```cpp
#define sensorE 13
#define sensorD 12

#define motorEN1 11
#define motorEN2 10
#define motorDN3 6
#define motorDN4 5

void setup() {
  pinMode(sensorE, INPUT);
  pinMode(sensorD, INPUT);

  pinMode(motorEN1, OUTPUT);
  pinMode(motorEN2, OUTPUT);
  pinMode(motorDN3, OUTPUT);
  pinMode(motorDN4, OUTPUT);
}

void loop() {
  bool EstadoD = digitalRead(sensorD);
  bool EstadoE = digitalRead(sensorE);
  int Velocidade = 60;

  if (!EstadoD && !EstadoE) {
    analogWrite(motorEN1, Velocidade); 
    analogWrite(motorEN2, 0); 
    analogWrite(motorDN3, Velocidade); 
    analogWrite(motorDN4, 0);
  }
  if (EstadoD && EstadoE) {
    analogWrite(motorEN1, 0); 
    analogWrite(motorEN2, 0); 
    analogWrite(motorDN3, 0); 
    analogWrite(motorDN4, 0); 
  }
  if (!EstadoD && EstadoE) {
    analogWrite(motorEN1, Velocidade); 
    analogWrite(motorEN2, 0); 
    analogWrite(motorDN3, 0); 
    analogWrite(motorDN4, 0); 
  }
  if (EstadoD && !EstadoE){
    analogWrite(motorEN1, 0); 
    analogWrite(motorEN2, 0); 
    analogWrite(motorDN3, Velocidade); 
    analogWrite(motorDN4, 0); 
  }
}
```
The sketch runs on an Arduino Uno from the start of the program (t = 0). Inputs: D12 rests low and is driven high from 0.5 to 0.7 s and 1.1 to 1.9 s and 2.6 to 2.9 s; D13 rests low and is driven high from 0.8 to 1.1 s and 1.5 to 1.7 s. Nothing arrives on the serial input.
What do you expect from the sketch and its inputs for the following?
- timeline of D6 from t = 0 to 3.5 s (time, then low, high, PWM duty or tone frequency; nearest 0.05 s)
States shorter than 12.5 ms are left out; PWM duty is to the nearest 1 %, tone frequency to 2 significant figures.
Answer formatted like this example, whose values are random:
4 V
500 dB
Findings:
0 s PWM 24 %; 0.8 s low; 1.1 s PWM 24 %; 1.5 s low; 1.7 s PWM 24 %
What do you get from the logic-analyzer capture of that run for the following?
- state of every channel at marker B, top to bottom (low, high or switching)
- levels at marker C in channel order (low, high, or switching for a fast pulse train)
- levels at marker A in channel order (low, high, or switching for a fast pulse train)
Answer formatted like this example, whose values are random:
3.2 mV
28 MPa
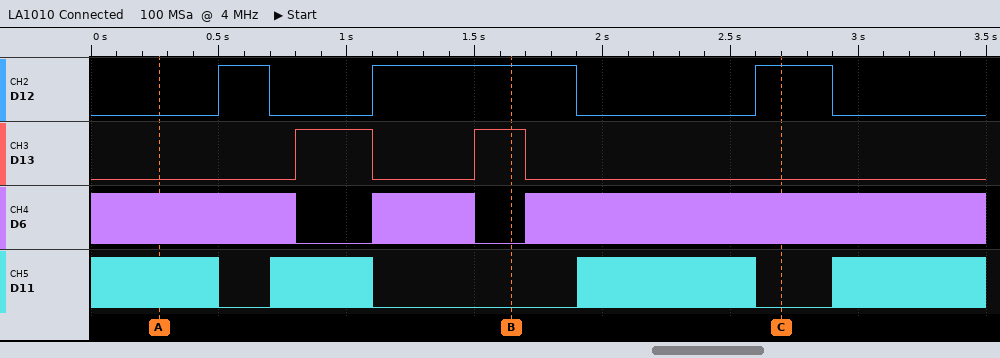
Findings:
D12 high, D13 high, D6 low, D11 low
D12 high, D13 low, D6 switching, D11 low
D12 low, D13 low, D6 switching, D11 switching
